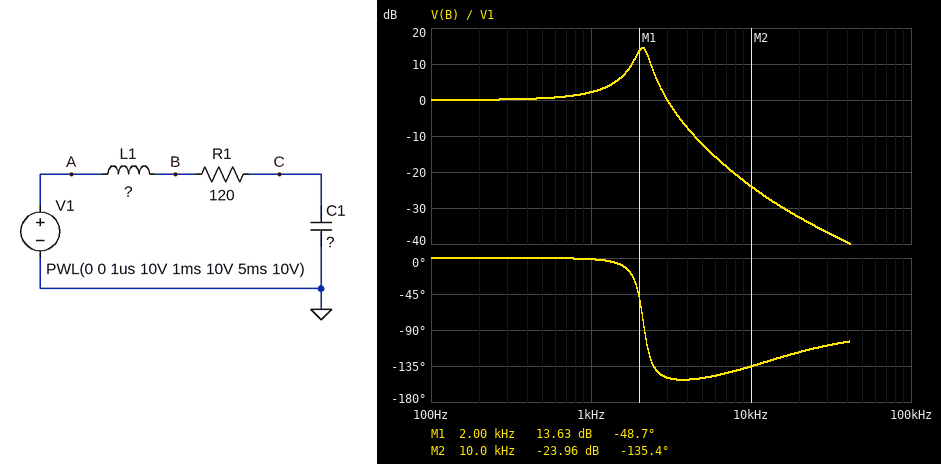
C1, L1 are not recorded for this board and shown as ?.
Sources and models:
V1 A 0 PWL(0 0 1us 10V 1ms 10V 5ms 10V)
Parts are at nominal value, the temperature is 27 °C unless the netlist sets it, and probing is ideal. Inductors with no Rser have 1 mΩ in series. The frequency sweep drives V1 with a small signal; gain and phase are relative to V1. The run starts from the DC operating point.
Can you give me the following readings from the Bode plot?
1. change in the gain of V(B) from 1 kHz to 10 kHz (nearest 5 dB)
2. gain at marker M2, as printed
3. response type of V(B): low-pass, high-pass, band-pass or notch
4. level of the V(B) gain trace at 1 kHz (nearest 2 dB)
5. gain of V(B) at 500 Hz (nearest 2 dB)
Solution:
-25 dB
-23.96 dB
low-pass
2 dB
0 dB
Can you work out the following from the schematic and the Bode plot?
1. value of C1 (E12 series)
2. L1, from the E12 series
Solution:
120 nF
47 mH
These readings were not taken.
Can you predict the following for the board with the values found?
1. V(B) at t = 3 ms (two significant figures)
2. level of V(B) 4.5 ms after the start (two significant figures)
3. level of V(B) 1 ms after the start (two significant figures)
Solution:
10 V
10 V
8.0 V
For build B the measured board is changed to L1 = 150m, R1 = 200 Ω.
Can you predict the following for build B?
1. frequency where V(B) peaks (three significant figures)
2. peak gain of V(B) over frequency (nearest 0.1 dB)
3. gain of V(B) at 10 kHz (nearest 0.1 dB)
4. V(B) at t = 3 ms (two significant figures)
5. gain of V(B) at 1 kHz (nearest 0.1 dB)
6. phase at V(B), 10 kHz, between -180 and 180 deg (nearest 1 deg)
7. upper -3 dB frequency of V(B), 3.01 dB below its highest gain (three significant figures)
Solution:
1.18 kHz
15.1 dB
-31.8 dB
11 V
9.8 dB
-122 deg
1.28 kHz
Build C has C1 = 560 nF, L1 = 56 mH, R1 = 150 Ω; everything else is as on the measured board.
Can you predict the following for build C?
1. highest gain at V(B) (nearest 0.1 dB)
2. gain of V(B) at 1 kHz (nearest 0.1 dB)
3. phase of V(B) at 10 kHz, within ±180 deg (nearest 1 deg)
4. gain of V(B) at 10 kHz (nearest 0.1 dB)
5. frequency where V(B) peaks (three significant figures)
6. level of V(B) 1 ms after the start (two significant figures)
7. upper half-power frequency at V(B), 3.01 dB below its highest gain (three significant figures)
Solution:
7.5 dB
5.8 dB
-98 deg
-27.2 dB
856 Hz
7.7 V
1.06 kHz
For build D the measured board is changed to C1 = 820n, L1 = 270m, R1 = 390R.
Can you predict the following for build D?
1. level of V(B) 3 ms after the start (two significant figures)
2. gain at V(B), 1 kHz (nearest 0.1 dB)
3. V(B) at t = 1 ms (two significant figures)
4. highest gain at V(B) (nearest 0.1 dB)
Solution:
8.8 V
-11.0 dB
14 V
5.3 dB
